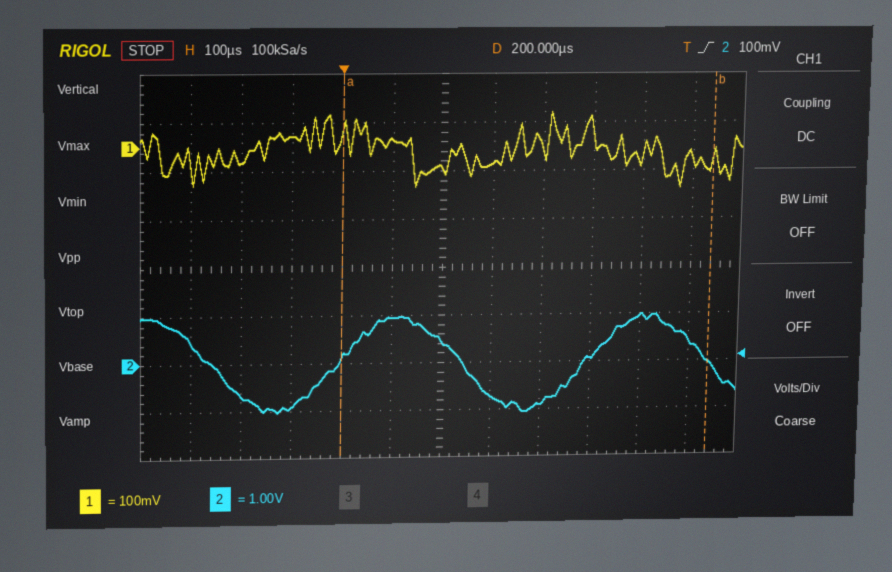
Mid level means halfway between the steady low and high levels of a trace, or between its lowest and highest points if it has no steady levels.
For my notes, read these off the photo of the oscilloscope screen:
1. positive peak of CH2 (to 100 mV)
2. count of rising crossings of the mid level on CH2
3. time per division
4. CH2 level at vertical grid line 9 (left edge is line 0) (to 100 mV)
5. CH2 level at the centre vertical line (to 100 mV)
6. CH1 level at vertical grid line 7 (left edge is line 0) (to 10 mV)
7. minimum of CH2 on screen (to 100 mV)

1.0 V
2
100 µs
100 mV
500 mV
-30 mV
-1.0 V
